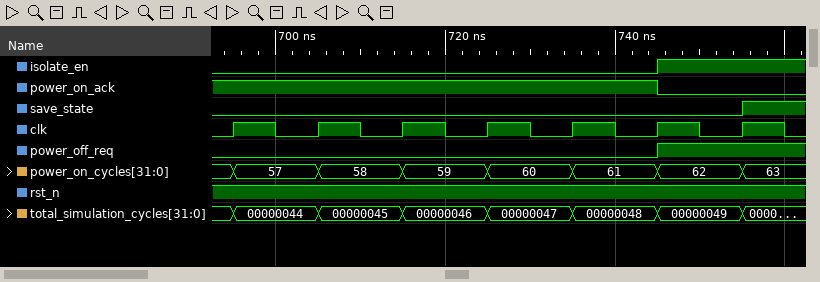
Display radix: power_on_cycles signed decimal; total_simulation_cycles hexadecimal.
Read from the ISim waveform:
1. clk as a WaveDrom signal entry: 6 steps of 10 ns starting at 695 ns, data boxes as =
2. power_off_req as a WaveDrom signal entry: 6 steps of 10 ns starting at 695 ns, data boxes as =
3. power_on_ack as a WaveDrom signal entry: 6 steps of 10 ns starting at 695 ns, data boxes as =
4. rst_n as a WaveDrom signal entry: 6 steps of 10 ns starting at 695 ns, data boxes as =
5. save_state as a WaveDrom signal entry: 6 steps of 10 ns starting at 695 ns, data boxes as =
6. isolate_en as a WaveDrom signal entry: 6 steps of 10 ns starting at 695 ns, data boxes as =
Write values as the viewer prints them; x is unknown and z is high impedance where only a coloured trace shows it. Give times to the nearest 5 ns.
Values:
{name: 'clk', wave: 'p.....'}
{name: 'power_off_req', wave: '0....1'}
{name: 'power_on_ack', wave: '1....0'}
{name: 'rst_n', wave: '1.....'}
{name: 'save_state', wave: '0.....'}
{name: 'isolate_en', wave: '0....1'}
